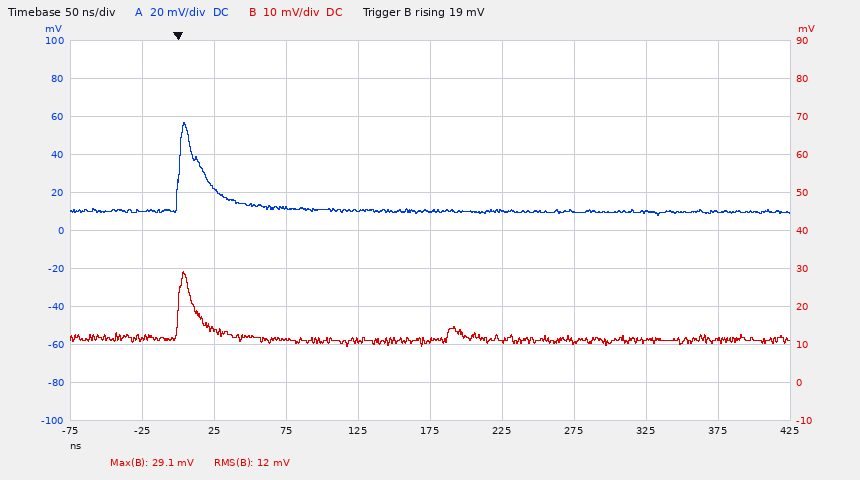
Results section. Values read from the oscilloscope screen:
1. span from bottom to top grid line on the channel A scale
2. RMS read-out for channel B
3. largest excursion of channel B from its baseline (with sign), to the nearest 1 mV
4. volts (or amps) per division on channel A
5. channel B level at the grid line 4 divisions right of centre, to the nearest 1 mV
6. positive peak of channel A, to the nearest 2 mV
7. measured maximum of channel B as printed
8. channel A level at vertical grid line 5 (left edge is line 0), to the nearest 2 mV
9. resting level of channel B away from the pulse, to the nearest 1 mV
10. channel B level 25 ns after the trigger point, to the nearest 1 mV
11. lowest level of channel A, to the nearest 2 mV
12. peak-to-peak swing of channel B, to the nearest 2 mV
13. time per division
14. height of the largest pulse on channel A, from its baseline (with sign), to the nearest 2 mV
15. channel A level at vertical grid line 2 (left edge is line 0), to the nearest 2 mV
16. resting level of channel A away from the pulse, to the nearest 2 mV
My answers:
200 mV
12 mV
+18 mV
20 mV
11 mV
56 mV
29.1 mV
10 mV
11 mV
14 mV
8 mV
20 mV
50 ns
+46 mV
22 mV
10 mV
